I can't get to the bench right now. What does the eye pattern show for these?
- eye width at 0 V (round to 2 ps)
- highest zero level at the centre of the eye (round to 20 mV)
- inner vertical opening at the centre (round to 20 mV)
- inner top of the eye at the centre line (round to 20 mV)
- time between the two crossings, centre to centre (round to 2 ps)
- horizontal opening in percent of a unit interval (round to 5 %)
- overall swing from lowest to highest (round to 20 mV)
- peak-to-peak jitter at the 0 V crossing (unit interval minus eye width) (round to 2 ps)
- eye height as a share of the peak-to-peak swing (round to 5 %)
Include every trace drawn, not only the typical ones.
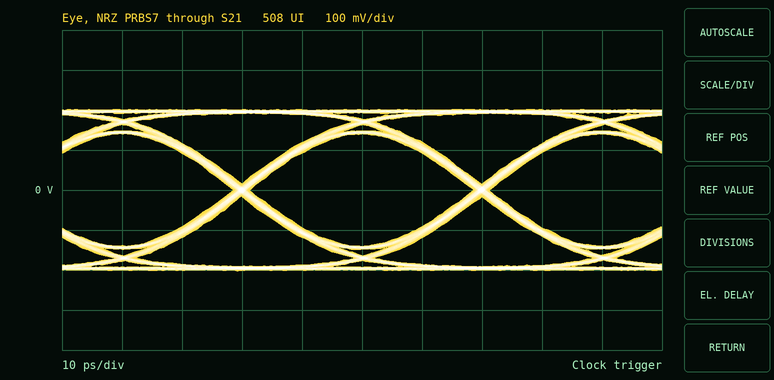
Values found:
38 ps
-140 mV
280 mV
140 mV
40 ps
95 %
400 mV
2 ps
70 %
